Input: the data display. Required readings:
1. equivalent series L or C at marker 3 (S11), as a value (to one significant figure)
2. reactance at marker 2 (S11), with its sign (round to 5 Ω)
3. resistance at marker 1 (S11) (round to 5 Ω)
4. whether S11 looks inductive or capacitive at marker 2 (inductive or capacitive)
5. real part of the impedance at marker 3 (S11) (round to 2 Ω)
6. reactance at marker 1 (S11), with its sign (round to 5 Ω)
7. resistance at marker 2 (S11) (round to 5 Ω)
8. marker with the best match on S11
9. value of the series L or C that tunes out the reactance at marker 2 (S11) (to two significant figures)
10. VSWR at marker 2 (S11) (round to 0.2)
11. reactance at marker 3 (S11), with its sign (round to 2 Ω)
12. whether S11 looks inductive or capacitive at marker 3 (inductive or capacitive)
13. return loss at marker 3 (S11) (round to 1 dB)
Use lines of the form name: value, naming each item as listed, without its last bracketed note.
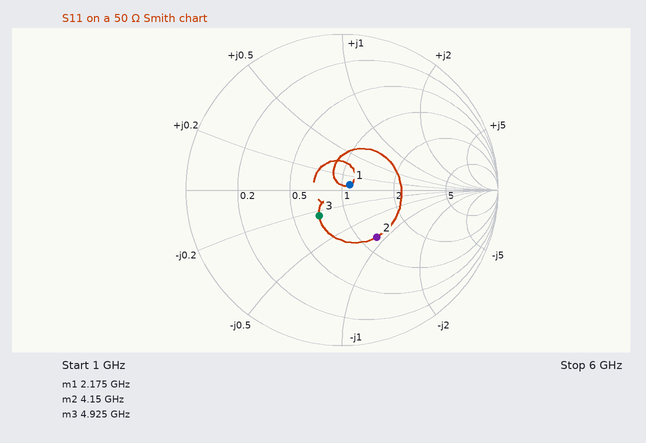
equivalent series L or C at marker 3 (S11), as a value: 3 pF
reactance at marker 2 (S11), with its sign: -45 Ω
resistance at marker 1 (S11): 55 Ω
whether S11 looks inductive or capacitive at marker 2: capacitive
real part of the impedance at marker 3 (S11): 36 Ω
reactance at marker 1 (S11), with its sign: +5 Ω
resistance at marker 2 (S11): 60 Ω
marker with the best match on S11: marker 1
value of the series L or C that tunes out the reactance at marker 2 (S11): 1.7 nH
VSWR at marker 2 (S11): 2.2
reactance at marker 3 (S11), with its sign: -12 Ω
whether S11 looks inductive or capacitive at marker 3: capacitive
return loss at marker 3 (S11): 13 dB
